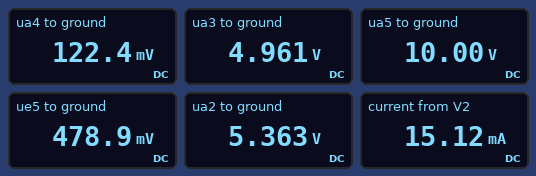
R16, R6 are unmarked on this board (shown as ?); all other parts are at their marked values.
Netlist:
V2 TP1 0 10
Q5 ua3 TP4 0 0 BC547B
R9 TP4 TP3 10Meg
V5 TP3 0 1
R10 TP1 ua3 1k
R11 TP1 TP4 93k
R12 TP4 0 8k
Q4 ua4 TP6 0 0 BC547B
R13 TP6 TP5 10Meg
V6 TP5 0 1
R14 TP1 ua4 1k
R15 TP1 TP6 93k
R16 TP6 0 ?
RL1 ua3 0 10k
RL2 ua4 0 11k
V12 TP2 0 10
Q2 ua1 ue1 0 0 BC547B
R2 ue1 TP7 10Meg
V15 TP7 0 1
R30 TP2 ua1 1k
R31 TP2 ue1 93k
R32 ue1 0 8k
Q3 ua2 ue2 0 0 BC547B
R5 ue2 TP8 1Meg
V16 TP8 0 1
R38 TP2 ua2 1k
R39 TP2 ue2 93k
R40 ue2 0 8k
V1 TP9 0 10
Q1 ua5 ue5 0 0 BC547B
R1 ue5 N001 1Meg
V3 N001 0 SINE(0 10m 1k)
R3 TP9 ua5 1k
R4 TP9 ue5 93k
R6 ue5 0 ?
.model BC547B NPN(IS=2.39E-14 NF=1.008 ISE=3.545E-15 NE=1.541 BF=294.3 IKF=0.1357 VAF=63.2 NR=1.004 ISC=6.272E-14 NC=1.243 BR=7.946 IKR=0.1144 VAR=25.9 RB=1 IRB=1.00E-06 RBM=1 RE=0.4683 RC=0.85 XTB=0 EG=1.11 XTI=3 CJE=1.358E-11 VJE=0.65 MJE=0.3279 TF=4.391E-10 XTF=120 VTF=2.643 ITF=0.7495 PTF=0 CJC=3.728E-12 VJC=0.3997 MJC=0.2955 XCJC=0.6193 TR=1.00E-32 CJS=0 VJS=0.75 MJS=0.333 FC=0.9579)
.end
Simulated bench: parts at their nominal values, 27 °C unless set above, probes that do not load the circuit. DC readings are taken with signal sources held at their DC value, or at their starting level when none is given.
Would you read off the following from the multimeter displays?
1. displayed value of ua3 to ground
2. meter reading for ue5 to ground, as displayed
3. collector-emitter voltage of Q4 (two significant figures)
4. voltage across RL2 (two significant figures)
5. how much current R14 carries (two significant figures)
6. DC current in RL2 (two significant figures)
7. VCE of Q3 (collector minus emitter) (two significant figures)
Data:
4.961 V
478.9 mV
120 mV
120 mV
9.9 mA
11 µA
5.4 V
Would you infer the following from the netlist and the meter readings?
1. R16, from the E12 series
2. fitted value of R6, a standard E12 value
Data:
22 kΩ
4.7 kΩ
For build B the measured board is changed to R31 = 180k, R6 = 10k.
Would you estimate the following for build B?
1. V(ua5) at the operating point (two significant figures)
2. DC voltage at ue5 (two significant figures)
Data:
1.9 V
700 mV
